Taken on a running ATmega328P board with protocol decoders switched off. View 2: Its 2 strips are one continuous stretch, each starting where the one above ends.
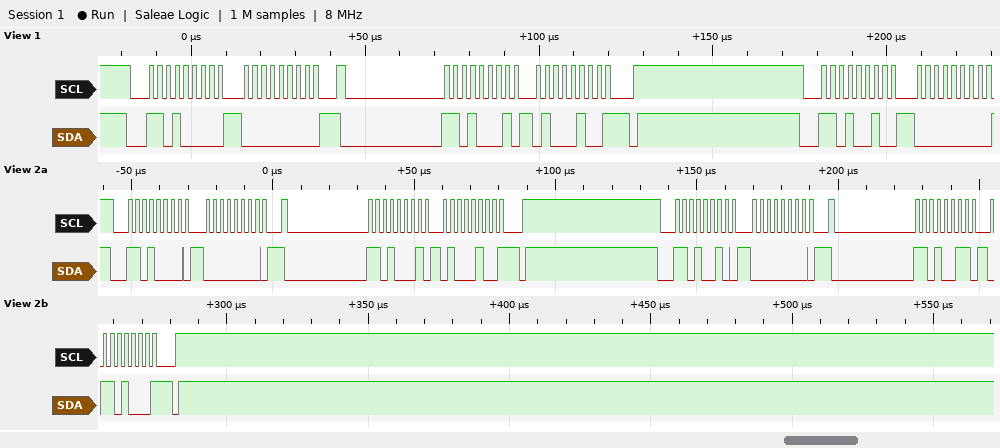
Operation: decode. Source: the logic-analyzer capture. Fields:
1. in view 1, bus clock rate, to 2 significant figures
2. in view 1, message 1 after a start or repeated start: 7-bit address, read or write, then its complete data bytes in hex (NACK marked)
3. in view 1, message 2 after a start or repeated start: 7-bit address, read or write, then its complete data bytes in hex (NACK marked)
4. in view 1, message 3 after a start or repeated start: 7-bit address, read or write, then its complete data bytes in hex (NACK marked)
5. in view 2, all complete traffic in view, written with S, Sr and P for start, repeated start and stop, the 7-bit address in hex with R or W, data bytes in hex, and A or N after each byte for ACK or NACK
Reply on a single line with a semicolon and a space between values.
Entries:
400 kHz; 0x68 write: 00; 0x68 read: 44 NACK; 0x69 write: 00; S 68W A 00 A Sr 68R A 44 N P S 69W A 00 A Sr 69R A 68 N P
